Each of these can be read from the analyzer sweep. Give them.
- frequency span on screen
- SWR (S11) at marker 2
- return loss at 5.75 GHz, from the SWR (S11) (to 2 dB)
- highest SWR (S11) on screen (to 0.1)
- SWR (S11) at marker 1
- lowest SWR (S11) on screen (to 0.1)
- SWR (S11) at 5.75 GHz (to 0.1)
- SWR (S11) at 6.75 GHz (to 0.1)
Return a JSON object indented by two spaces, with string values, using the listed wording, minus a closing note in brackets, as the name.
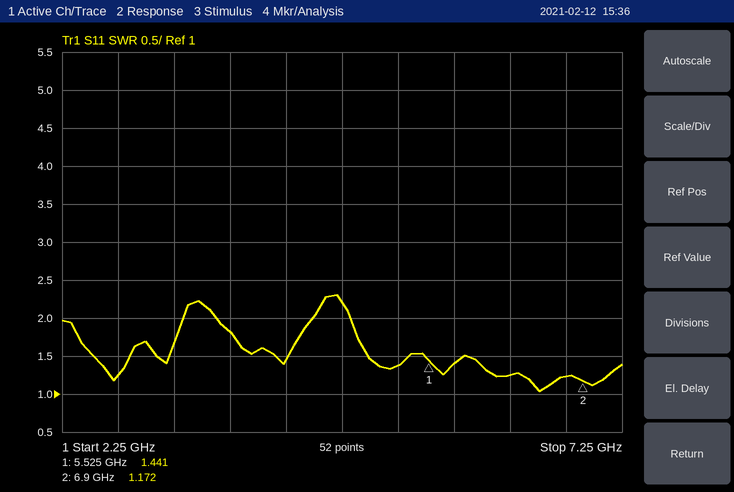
{
  "frequency span on screen": "5 GHz",
  "SWR (S11) at marker 2": "1.172",
  "return loss at 5.75 GHz, from the SWR (S11)": "16 dB",
  "highest SWR (S11) on screen": "2.3",
  "SWR (S11) at marker 1": "1.441",
  "lowest SWR (S11) on screen": "1.0",
  "SWR (S11) at 5.75 GHz": "1.4",
  "SWR (S11) at 6.75 GHz": "1.2"
}
